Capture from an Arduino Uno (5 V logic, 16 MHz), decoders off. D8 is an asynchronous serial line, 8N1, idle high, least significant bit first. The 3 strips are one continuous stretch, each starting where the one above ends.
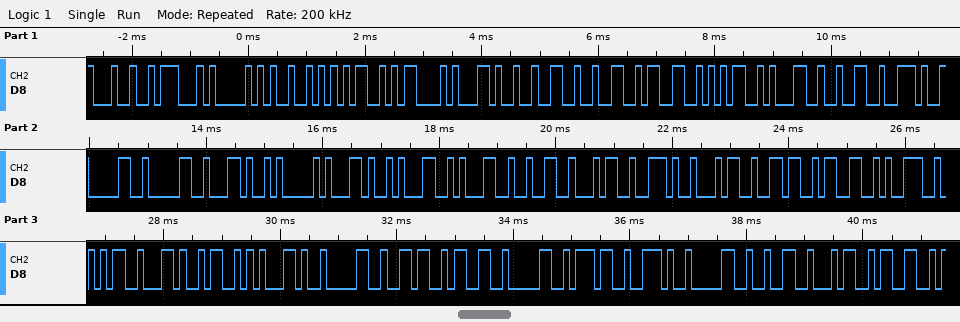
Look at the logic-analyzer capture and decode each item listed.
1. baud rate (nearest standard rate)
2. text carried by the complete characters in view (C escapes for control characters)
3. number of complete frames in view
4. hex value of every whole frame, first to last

9600 baud
"$GPRMC,223512.00,A,1124.46395,S,06307.0243"
42
24 47 50 52 4D 43 2C 32 32 33 35 31 32 2E 30 30 2C 41 2C 31 31 32 34 2E 34 36 33 39 35 2C 53 2C 30 36 33 30 37 2E 30 32 34 33
